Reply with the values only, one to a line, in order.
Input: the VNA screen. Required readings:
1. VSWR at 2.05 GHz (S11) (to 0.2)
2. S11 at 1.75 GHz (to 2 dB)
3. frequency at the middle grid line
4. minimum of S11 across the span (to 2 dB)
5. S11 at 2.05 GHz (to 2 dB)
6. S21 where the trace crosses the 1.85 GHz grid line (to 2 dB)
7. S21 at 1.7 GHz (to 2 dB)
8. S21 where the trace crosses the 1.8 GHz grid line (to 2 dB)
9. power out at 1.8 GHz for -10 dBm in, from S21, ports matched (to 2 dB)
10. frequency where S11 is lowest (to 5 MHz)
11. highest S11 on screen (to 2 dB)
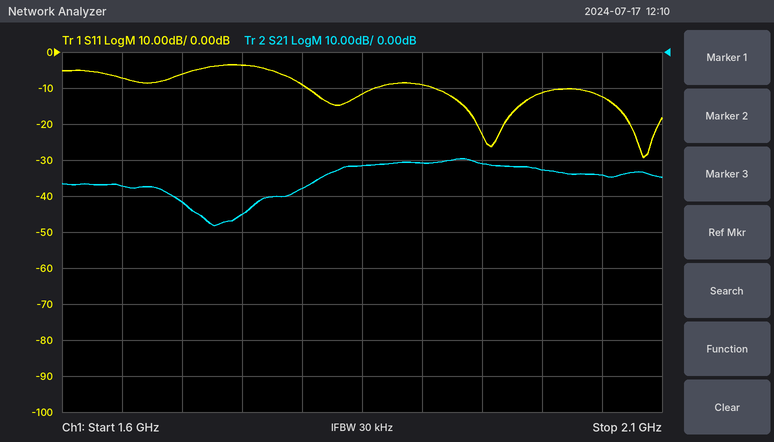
1.6
-4 dB
1.85 GHz
-30 dB
-12 dB
-32 dB
-42 dB
-38 dB
-48 dBm
2.085 GHz
-4 dB
